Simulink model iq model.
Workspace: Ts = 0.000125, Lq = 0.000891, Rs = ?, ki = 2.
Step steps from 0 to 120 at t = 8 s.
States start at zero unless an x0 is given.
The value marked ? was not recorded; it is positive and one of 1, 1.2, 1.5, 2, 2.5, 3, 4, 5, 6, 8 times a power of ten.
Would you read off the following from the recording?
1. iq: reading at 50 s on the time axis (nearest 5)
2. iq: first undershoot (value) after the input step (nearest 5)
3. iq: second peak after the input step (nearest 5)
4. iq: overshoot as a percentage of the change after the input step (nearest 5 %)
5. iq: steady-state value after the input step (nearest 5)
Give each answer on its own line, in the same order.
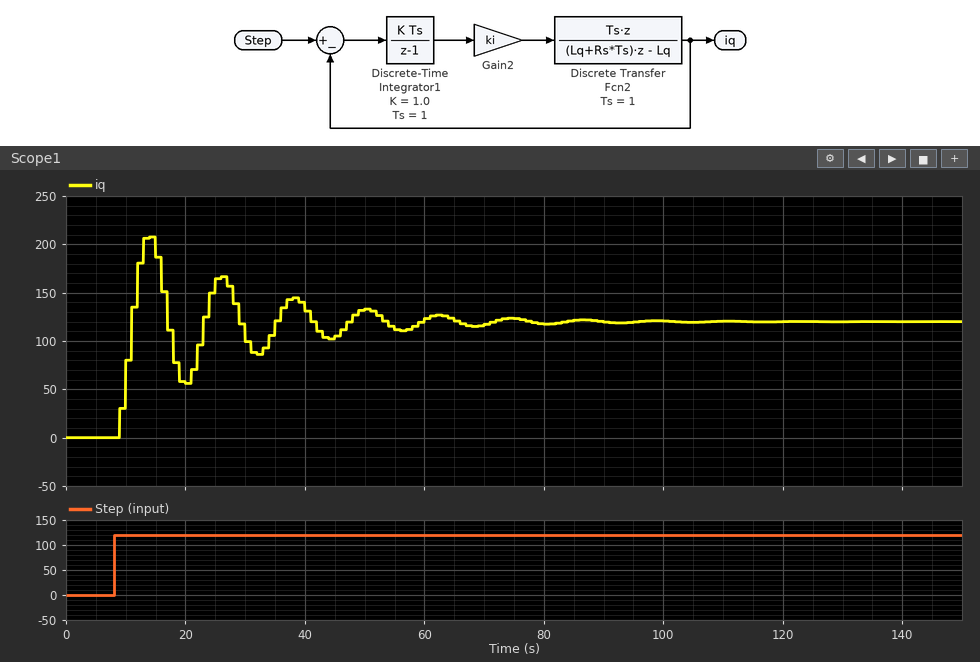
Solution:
135
55
165
75 %
120
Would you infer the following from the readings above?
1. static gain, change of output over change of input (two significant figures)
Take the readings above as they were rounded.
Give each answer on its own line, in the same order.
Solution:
1.0
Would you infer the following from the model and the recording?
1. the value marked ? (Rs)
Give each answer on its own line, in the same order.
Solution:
0.8
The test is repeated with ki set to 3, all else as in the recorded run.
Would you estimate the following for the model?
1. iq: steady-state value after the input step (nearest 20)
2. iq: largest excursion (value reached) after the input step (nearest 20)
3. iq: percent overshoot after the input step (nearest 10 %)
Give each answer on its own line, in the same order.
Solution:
120
220
80 %
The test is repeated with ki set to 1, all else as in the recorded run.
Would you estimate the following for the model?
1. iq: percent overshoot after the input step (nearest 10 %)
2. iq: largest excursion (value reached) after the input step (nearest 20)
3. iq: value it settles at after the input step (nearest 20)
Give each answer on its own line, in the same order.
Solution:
60 %
200
120
